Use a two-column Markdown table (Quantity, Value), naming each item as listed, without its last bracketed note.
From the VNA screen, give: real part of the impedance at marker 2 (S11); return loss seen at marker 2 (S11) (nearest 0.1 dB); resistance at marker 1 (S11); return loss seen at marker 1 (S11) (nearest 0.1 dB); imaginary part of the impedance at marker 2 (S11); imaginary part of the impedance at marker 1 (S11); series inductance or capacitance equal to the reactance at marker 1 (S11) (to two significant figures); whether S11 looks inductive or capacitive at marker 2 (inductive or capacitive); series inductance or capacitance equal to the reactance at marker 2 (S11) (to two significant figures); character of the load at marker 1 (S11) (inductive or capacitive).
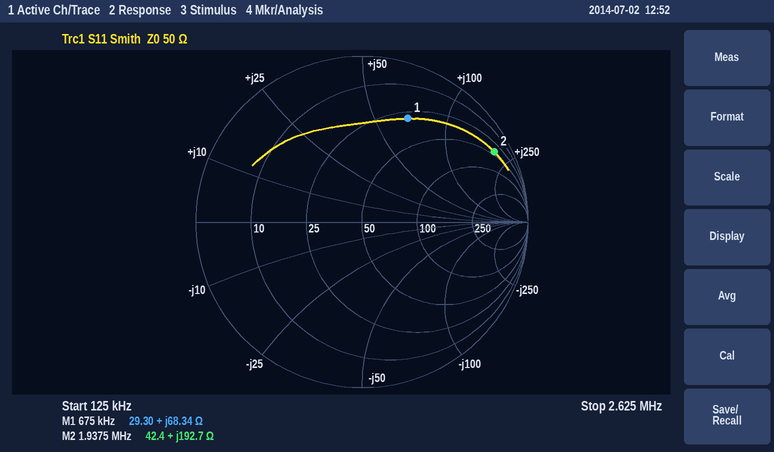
| Quantity | Value |
|---|---|
| real part of the impedance at marker 2 | 42.4 Ω |
| return loss seen at marker 2 (S11) | 0.9 dB |
| resistance at marker 1 | 29.30 Ω |
| return loss seen at marker 1 (S11) | 3.3 dB |
| imaginary part of the impedance at marker 2 | +192.7 Ω |
| imaginary part of the impedance at marker 1 | +68.34 Ω |
| series inductance or capacitance equal to the reactance at marker 1 (S11) | 16 µH |
| whether S11 looks inductive or capacitive at marker 2 | inductive |
| series inductance or capacitance equal to the reactance at marker 2 (S11) | 16 µH |
| character of the load at marker 1 (S11) | inductive |
